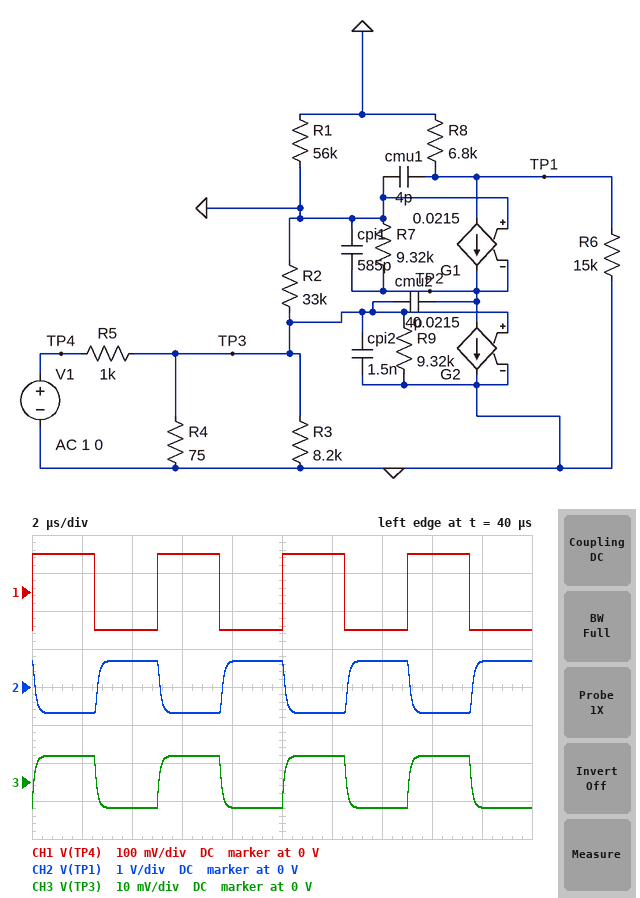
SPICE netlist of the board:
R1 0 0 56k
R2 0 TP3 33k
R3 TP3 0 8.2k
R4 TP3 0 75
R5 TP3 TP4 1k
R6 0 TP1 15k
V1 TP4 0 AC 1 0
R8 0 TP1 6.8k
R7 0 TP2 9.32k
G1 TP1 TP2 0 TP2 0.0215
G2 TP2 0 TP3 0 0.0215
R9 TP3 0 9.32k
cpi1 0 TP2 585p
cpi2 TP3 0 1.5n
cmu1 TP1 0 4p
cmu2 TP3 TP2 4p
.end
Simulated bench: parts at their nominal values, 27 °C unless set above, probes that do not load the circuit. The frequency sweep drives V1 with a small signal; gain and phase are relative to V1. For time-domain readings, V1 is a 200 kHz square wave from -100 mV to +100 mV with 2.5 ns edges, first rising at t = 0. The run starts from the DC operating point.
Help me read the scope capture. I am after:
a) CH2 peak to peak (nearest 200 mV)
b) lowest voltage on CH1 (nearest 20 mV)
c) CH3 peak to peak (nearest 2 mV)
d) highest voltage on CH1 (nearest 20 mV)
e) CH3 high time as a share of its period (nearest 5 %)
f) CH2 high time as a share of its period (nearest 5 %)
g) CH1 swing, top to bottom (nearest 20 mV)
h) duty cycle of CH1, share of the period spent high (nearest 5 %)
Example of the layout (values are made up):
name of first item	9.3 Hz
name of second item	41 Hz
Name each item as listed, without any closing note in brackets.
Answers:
CH2 peak to peak	1.4 V
lowest voltage on CH1	-100 mV
CH3 peak to peak	14 mV
highest voltage on CH1	100 mV
CH3 high time as a share of its period	50 %
CH2 high time as a share of its period	50 %
CH1 swing, top to bottom	200 mV
duty cycle of CH1, share of the period spent high	50 %
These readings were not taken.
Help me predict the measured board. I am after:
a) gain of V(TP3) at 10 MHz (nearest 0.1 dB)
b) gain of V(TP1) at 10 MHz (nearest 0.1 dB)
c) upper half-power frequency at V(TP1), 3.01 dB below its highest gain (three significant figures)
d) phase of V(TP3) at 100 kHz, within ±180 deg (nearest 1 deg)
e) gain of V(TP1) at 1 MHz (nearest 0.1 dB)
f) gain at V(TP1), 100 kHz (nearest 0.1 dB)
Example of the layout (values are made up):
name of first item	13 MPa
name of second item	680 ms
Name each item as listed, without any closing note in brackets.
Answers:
gain of V(TP3) at 10 MHz	-39.6 dB
gain of V(TP1) at 10 MHz	-9.3 dB
upper half-power frequency at V(TP1), 3.01 dB below its highest gain	1.41 MHz
phase of V(TP3) at 100 kHz, within ±180 deg	-4 deg
gain of V(TP1) at 1 MHz	15.0 dB
gain at V(TP1), 100 kHz	16.7 dB
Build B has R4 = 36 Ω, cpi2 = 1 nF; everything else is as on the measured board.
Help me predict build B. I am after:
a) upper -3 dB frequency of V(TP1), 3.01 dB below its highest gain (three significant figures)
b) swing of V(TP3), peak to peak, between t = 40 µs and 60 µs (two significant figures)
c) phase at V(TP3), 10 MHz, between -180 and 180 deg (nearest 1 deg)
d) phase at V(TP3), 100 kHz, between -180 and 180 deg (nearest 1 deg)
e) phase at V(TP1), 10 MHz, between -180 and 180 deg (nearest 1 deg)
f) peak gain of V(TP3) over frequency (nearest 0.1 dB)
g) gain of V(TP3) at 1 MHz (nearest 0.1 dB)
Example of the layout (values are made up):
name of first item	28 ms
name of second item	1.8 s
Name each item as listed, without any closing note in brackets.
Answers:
upper -3 dB frequency of V(TP1), 3.01 dB below its highest gain	2.96 MHz
swing of V(TP3), peak to peak, between t = 40 µs and 60 µs	6.9 mV
phase at V(TP3), 10 MHz, between -180 and 180 deg	-65 deg
phase at V(TP3), 100 kHz, between -180 and 180 deg	-1 deg
phase at V(TP1), 10 MHz, between -180 and 180 deg	5 deg
peak gain of V(TP3) over frequency	-29.3 dB
gain of V(TP3) at 1 MHz	-29.5 dB
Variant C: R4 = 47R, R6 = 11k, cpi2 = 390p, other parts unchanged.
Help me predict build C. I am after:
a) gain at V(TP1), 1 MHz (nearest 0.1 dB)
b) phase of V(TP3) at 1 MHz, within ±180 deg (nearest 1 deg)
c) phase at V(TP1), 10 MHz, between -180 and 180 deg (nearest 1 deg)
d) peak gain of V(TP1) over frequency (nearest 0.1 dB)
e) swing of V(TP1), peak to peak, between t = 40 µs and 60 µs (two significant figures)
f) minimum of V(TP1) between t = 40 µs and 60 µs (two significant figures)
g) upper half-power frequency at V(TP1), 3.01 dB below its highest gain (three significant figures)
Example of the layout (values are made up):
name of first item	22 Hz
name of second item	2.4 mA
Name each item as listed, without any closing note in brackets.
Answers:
gain at V(TP1), 1 MHz	11.8 dB
phase of V(TP3) at 1 MHz, within ±180 deg	-6 deg
phase at V(TP1), 10 MHz, between -180 and 180 deg	25 deg
peak gain of V(TP1) over frequency	12.0 dB
swing of V(TP1), peak to peak, between t = 40 µs and 60 µs	800 mV
minimum of V(TP1) between t = 40 µs and 60 µs	-400 mV
upper half-power frequency at V(TP1), 3.01 dB below its highest gain	3.88 MHz
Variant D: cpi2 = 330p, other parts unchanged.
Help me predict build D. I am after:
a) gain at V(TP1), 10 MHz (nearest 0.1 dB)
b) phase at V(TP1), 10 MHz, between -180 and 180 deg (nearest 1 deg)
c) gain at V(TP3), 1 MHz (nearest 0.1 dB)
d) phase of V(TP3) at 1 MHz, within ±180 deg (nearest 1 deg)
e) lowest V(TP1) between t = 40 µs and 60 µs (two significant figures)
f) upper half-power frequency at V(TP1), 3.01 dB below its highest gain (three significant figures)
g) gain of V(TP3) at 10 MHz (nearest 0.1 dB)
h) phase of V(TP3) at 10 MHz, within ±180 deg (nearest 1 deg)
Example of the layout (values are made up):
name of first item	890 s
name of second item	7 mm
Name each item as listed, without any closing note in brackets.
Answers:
gain at V(TP1), 10 MHz	2.1 dB
phase at V(TP1), 10 MHz, between -180 and 180 deg	15 deg
gain at V(TP3), 1 MHz	-23.4 dB
phase of V(TP3) at 1 MHz, within ±180 deg	-8 deg
lowest V(TP1) between t = 40 µs and 60 µs	-690 mV
upper half-power frequency at V(TP1), 3.01 dB below its highest gain	3.49 MHz
gain of V(TP3) at 10 MHz	-28.2 dB
phase of V(TP3) at 10 MHz, within ±180 deg	-55 deg
